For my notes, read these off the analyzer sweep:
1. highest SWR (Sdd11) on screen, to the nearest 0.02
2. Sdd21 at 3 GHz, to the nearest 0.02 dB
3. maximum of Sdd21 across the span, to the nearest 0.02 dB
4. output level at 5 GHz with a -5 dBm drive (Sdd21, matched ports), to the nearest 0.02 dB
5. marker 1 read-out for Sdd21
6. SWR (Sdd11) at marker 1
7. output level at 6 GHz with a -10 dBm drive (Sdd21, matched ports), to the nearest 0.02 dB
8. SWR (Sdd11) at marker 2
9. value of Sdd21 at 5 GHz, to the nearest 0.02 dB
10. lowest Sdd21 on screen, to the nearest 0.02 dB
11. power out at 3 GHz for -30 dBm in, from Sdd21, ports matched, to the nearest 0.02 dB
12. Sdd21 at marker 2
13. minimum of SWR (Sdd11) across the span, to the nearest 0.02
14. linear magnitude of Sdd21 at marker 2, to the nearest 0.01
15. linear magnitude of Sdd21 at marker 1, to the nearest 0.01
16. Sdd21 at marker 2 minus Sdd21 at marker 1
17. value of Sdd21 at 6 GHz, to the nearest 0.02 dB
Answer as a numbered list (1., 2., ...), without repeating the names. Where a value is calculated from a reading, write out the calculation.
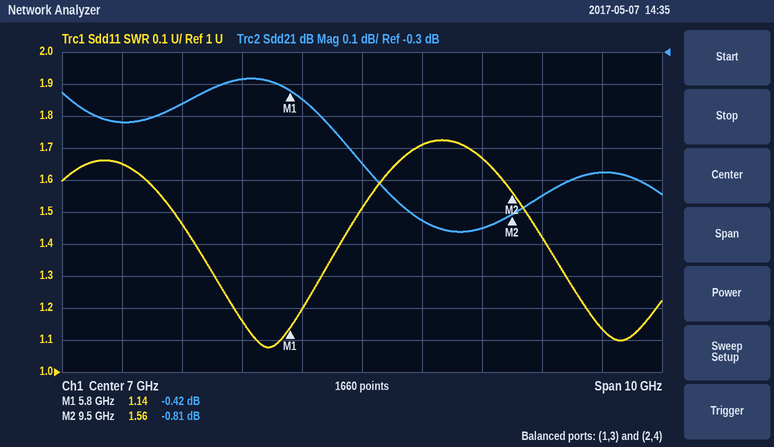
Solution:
1. 1.72
2. -0.52 dB
3. -0.38 dB
4. -5 dBm + (-0.38 dB) = -5.38 dBm
5. -0.42 dB
6. 1.14
7. -10 dBm + (-0.44 dB) = -10.44 dBm
8. 1.56
9. -0.38 dB
10. -0.86 dB
11. -30 dBm + (-0.52 dB) = -30.52 dBm
12. -0.81 dB
13. 1.08
14. 10^(-0.81/20) ≈ 0.91
15. 10^(-0.42/20) ≈ 0.95
16. -0.81 − (-0.42) = -0.39 dB
17. -0.44 dB
